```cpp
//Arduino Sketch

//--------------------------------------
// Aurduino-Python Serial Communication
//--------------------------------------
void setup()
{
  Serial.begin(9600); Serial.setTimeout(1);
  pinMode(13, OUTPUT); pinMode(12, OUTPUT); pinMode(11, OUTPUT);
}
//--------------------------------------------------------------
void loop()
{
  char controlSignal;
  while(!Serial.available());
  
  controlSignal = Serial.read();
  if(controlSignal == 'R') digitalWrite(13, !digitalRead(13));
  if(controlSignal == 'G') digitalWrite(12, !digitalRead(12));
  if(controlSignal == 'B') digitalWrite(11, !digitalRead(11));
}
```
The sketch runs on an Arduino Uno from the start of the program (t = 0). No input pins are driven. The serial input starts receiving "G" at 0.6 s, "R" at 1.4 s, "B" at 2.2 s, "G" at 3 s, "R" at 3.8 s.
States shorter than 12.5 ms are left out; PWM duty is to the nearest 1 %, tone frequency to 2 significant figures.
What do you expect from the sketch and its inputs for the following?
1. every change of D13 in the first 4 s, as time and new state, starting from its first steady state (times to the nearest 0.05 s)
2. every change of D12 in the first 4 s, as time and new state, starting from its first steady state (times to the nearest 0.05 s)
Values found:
0 s low; 1.4 s high; 3.8 s low
0 s low; 0.6 s high; 3 s low
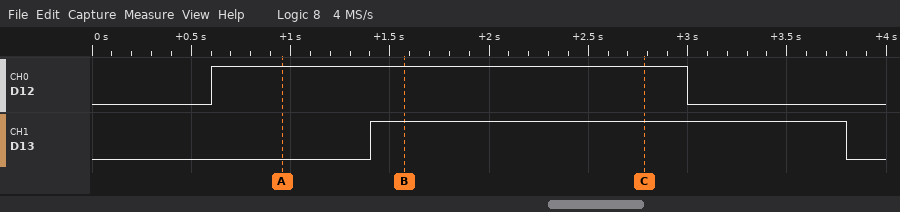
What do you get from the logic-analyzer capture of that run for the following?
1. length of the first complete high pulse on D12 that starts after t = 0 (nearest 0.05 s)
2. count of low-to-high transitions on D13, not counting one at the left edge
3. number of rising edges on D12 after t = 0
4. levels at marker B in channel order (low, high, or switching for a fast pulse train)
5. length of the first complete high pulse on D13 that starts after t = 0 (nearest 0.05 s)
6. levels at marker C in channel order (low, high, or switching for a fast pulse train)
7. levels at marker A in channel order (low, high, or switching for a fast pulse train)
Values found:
2.40 s
1
1
D12 high, D13 high
2.40 s
D12 high, D13 high
D12 high, D13 low
